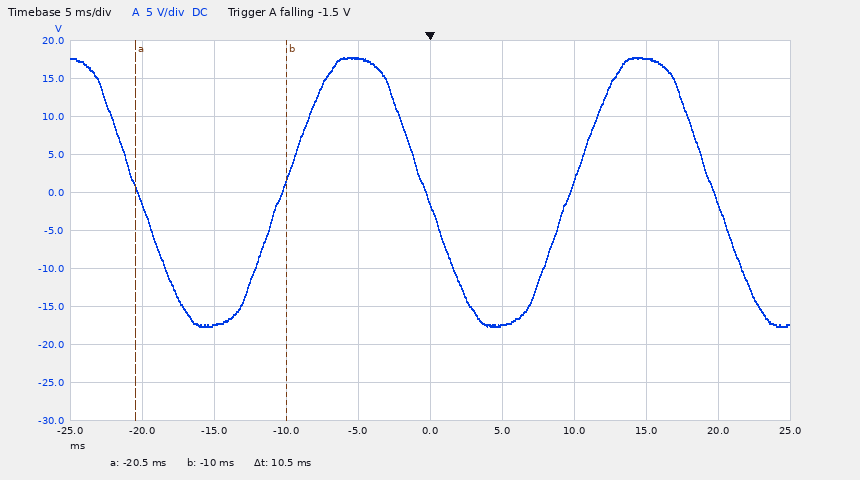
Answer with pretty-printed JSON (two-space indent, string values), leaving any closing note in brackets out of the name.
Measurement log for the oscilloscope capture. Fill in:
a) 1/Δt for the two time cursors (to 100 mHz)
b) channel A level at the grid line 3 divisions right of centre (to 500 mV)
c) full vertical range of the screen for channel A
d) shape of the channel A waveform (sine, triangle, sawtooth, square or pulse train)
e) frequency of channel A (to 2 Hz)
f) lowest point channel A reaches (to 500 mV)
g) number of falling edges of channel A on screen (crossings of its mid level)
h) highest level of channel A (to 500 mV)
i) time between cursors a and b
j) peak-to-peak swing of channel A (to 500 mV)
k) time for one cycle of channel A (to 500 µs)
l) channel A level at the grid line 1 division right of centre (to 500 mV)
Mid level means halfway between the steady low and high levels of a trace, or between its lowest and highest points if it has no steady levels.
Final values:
{
  "1/Δt for the two time cursors": "95.2 Hz",
  "channel A level at the grid line 3 divisions right of centre": "17.5 V",
  "full vertical range of the screen for channel A": "50 V",
  "shape of the channel A waveform": "sine",
  "frequency of channel A": "50 Hz",
  "lowest point channel A reaches": "-17.5 V",
  "number of falling edges of channel A on screen": "3",
  "highest level of channel A": "18.0 V",
  "time between cursors a and b": "10.5 ms",
  "peak-to-peak swing of channel A": "35.5 V",
  "time for one cycle of channel A": "20.0 ms",
  "channel A level at the grid line 1 division right of centre": "-17.5 V"
}
